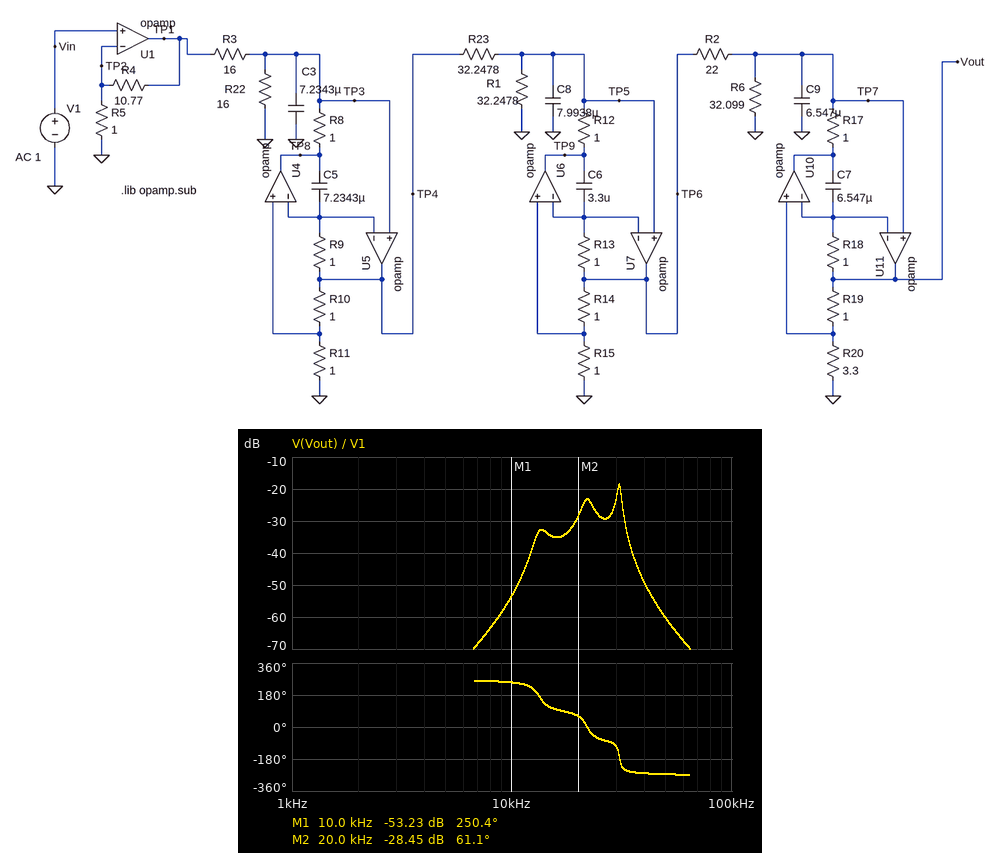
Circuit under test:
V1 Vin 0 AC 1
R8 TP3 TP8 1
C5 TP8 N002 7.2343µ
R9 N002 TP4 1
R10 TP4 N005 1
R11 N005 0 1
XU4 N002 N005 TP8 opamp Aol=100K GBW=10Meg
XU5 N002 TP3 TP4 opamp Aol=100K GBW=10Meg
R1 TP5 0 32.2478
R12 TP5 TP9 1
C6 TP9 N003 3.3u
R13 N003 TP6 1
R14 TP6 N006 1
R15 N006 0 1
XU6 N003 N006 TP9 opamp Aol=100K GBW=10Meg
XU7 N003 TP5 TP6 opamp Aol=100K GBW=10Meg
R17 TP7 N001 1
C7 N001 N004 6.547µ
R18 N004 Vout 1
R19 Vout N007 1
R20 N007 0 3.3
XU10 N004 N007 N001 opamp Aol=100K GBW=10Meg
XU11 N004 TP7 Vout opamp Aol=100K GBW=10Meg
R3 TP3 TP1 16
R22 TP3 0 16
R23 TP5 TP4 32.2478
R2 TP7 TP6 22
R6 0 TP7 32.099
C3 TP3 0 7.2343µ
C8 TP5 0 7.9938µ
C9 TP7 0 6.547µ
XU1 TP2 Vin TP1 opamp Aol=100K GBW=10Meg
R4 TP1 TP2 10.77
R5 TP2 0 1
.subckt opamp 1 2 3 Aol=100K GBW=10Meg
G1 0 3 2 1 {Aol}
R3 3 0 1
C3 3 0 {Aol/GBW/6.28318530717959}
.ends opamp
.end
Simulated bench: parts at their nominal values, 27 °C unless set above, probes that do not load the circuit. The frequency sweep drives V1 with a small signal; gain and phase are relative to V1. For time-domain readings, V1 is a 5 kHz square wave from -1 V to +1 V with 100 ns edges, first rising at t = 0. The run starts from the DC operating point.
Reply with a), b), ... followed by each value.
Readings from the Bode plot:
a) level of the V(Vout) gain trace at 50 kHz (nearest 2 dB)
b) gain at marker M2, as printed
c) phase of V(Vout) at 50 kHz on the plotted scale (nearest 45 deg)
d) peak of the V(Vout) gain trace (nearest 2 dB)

a) -60 dB
b) -28.45 dB
c) -270 deg
d) -18 dB
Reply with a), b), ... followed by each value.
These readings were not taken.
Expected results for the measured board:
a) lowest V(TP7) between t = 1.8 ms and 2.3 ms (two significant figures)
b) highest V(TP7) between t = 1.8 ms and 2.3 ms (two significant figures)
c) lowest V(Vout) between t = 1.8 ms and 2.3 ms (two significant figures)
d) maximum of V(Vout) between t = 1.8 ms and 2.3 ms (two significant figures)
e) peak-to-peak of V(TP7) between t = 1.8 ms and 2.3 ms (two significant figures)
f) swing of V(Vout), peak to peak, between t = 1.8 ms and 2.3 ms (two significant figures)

a) -14 mV
b) 14 mV
c) -18 mV
d) 18 mV
e) 28 mV
f) 36 mV
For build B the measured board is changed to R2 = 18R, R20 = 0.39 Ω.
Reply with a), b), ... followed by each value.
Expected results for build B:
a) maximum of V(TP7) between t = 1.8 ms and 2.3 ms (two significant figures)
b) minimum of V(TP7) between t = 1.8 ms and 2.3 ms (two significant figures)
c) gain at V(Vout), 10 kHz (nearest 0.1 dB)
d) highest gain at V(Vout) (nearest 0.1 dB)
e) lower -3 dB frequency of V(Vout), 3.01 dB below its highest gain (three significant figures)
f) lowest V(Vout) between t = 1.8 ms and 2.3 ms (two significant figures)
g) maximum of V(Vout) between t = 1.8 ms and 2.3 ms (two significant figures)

a) 12 mV
b) -12 mV
c) -67.6 dB
d) -5.1 dB
e) 30.2 kHz
f) -44 mV
g) 44 mV
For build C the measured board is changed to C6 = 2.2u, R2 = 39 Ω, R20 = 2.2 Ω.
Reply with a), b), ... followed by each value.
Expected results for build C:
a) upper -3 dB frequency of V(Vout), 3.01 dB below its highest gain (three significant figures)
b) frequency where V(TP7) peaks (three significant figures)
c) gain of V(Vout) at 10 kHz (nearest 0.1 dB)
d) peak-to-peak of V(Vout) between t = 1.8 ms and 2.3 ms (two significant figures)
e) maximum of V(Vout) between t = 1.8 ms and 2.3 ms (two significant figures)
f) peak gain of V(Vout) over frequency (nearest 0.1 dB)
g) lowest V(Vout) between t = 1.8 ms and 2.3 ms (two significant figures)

a) 38.2 kHz
b) 37.6 kHz
c) -67.5 dB
d) 14 mV
e) 7.2 mV
f) -28.5 dB
g) -7.2 mV
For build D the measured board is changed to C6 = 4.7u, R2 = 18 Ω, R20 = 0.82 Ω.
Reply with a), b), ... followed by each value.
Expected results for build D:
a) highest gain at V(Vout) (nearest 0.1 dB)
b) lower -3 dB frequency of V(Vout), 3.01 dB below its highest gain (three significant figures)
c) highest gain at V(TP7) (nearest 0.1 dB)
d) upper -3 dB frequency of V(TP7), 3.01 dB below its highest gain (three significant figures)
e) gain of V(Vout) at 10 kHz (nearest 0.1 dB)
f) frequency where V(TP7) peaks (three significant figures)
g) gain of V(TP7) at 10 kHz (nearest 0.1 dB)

a) 13.2 dB
b) 25.4 kHz
c) 6.3 dB
d) 26.6 kHz
e) -61.1 dB
f) 25.9 kHz
g) -68.0 dB
